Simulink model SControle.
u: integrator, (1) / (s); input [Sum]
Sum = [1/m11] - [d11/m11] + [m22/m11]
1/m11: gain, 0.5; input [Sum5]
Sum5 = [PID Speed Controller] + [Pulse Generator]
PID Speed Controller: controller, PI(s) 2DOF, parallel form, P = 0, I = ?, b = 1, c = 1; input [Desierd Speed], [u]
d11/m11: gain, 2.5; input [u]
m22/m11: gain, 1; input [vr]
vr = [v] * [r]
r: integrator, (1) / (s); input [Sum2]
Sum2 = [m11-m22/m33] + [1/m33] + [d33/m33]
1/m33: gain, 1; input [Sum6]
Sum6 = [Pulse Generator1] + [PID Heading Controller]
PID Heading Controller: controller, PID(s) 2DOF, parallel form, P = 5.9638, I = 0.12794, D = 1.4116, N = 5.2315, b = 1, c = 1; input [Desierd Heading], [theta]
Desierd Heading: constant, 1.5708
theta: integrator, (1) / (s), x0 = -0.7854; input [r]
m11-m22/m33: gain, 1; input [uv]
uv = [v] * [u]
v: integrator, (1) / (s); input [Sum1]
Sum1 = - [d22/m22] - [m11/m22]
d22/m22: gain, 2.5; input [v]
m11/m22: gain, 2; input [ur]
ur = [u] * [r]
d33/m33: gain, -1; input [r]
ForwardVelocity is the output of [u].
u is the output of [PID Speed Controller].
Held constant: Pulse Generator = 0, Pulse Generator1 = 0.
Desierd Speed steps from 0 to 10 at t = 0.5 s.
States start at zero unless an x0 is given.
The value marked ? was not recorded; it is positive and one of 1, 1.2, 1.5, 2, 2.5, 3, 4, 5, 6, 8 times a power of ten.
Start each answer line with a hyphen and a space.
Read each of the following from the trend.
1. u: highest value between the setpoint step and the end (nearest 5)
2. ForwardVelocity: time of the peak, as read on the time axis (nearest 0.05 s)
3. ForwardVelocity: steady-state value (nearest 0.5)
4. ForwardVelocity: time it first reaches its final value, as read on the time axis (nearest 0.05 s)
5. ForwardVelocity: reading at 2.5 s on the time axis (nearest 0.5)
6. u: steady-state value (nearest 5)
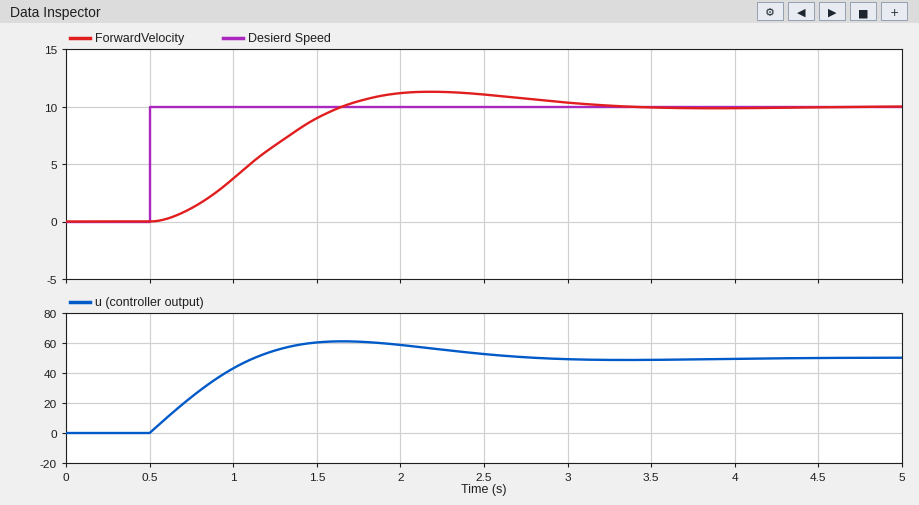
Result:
- 60
- 2.20 s
- 10.0
- 1.65 s
- 11.0
- 50
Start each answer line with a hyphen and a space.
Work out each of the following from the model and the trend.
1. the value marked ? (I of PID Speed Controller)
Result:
- 10
